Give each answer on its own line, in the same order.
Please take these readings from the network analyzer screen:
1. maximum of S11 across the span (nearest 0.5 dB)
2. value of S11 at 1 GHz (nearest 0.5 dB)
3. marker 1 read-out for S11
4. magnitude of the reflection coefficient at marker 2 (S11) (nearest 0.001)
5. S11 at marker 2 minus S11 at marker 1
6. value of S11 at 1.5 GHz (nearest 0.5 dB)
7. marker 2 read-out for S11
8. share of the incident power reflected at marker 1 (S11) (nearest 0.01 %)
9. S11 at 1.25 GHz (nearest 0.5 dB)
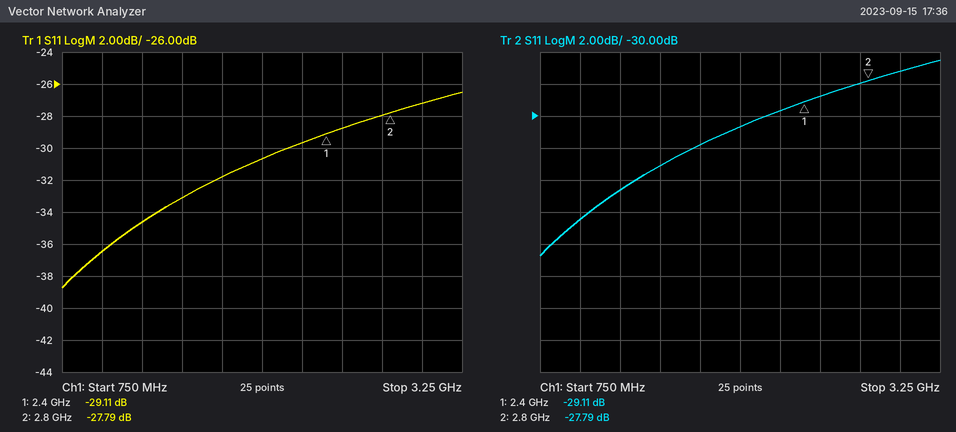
-26.5 dB
-36.5 dB
-29.11 dB
0.041
1.32 dB
-33.0 dB
-27.79 dB
0.12 %
-34.5 dB
